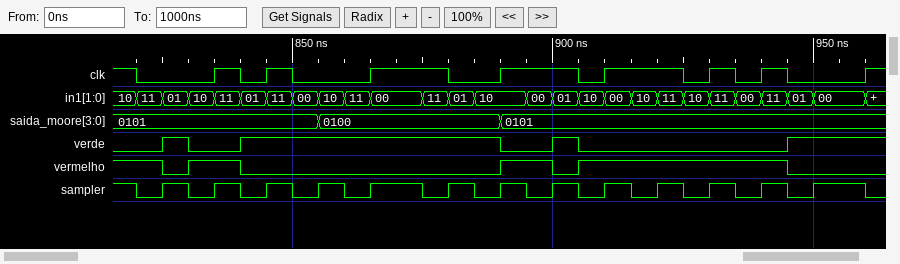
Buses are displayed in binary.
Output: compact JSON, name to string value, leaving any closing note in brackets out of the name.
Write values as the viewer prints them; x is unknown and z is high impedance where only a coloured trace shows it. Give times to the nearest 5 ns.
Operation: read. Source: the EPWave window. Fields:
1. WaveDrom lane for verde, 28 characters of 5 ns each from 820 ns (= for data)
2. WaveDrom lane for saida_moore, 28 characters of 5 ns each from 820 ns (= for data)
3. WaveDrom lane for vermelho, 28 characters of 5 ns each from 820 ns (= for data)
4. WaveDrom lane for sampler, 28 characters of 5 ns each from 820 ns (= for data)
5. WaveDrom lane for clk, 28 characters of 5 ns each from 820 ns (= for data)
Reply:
{"WaveDrom lane for verde, 28 characters of 5 ns each from 820 ns": "{name: 'verde', wave: '010.1.........0.10.......1..'}", "WaveDrom lane for saida_moore, 28 characters of 5 ns each from 820 ns": "{name: 'saida_moore', wave: '=......=......=.............', data: '0101 0100 0101'}", "WaveDrom lane for vermelho, 28 characters of 5 ns each from 820 ns": "{name: 'vermelho', wave: '101.0.........1.01.......0..'}", "WaveDrom lane for sampler, 28 characters of 5 ns each from 820 ns": "{name: 'sampler', wave: '0101010101.0101010101010101.'}", "WaveDrom lane for clk, 28 characters of 5 ns each from 820 ns": "{name: 'clk', wave: '0..1010..1..0.1..01..01010..'}"}
